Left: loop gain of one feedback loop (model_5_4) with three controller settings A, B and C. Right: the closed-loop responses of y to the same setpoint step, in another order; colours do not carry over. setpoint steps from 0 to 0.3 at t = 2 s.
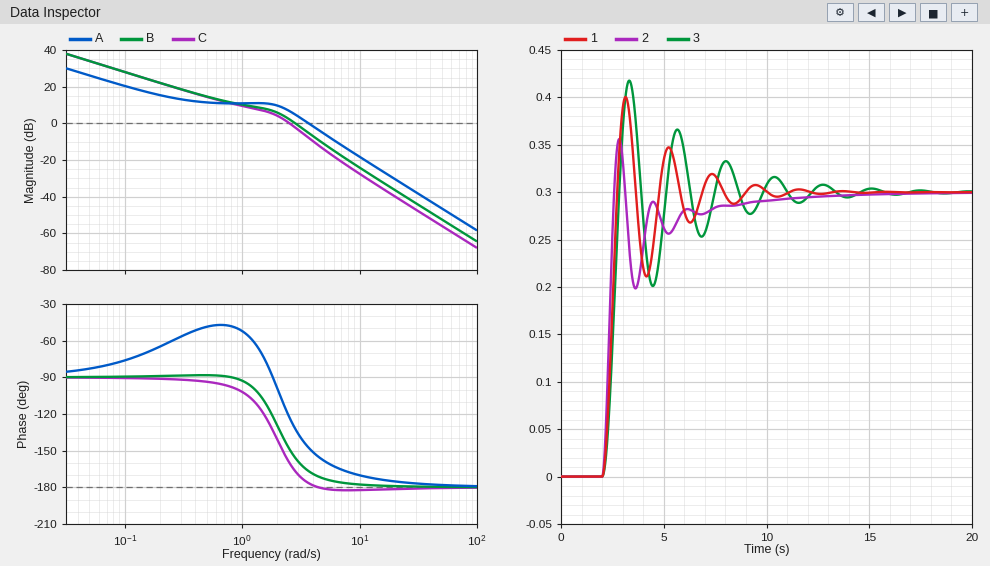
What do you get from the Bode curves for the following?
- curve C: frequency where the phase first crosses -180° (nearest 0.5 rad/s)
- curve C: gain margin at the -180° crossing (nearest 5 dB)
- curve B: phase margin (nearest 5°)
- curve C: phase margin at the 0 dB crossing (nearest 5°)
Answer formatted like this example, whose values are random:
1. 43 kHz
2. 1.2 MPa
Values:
1. 4.5 rad/s
2. 10 dB
3. 25°
4. 20°
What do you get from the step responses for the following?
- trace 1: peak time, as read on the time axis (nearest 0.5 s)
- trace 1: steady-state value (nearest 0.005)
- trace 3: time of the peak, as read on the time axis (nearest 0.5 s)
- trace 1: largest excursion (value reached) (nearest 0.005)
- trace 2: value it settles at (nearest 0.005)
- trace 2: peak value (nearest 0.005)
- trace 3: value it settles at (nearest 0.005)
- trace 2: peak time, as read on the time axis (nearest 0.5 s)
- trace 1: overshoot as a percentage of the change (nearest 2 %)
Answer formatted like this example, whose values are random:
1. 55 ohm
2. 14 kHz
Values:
1. 3.0 s
2. 0.300
3. 3.5 s
4. 0.400
5. 0.300
6. 0.355
7. 0.300
8. 3.0 s
9. 34 %
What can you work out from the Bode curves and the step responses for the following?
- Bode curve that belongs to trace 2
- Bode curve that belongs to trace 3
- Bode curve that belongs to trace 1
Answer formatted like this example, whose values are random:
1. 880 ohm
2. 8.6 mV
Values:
1. A
2. C
3. B
